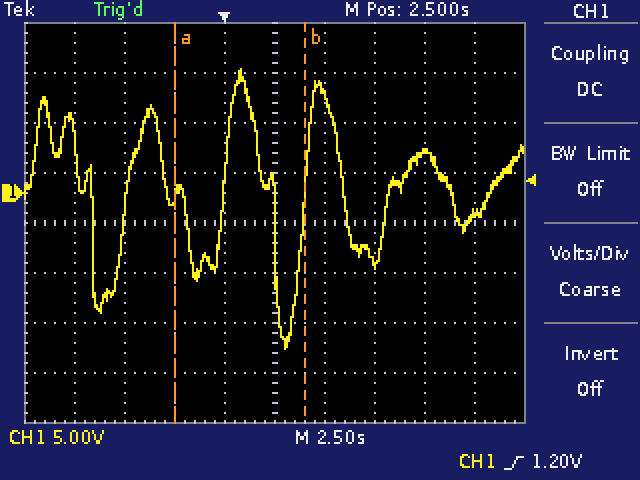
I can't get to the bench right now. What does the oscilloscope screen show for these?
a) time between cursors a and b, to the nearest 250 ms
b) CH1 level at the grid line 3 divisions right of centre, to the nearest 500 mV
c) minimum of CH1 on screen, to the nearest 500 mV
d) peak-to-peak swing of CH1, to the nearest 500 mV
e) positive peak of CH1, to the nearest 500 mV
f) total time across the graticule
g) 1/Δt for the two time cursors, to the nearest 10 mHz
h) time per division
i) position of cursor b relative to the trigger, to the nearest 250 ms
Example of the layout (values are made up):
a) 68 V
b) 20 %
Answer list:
a) 6.50 s
b) 4.0 V
c) -15.5 V
d) 28.0 V
e) 12.5 V
f) 25 s
g) 150 mHz
h) 2.5 s
i) +4.00 s
